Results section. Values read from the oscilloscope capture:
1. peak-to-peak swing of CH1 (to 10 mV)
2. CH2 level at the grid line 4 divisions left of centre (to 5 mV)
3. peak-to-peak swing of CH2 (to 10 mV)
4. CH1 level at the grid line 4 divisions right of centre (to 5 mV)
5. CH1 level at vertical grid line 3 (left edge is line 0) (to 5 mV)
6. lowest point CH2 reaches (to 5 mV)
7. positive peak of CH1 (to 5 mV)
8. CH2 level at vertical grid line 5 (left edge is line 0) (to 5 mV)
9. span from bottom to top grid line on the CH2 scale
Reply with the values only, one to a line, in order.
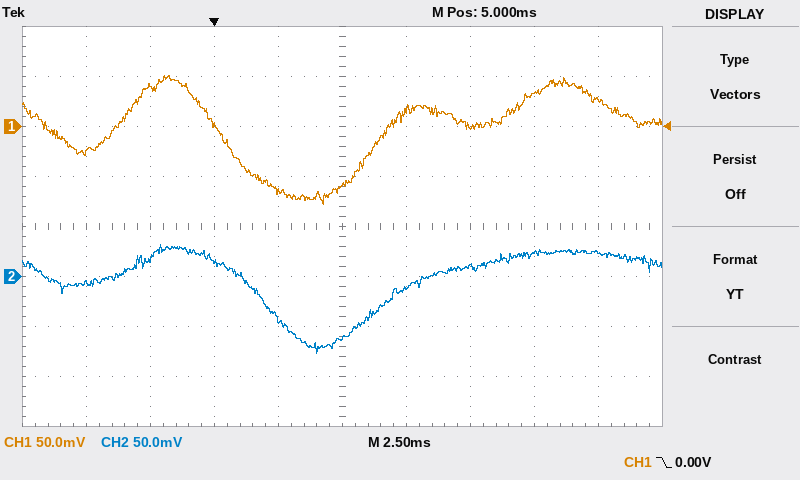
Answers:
130 mV
-5 mV
110 mV
25 mV
5 mV
-75 mV
50 mV
-60 mV
400 mV
